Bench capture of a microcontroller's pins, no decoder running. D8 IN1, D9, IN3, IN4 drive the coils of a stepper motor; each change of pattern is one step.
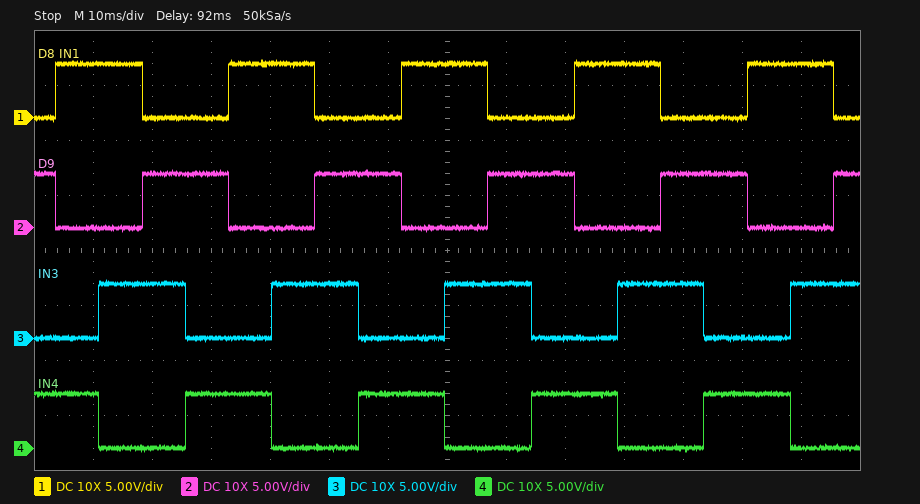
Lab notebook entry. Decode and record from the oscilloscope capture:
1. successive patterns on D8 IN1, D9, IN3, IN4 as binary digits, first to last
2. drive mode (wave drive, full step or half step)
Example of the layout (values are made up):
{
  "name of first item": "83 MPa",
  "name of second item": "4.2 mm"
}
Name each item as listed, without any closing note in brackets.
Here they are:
{
  "successive patterns on D8 IN1, D9, IN3, IN4 as binary digits, first to last": "0101 1001 1010 0110 0101 1001 1010 0110 0101 1001 1010 0110 0101 1001 1010 0110 0101 1001 1010 0110",
  "drive mode": "full step"
}
